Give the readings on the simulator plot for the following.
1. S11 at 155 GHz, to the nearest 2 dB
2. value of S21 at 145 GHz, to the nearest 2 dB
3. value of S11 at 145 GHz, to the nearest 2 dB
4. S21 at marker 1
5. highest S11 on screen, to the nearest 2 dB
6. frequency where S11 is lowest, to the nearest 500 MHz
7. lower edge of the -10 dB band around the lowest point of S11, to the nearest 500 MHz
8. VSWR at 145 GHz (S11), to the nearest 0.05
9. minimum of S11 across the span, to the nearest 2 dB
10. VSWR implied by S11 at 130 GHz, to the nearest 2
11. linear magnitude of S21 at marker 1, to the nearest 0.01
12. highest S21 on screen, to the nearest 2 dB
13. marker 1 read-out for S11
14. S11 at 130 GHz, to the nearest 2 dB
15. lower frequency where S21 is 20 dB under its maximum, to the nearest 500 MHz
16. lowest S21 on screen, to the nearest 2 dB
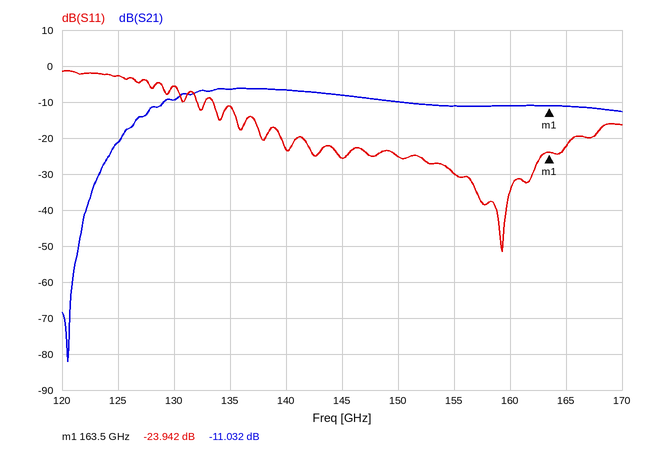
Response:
-30 dB
-8 dB
-26 dB
-11.032 dB
-2 dB
159.5 GHz
133.5 GHz
1.10
-52 dB
4
0.28
-6 dB
-23.942 dB
-6 dB
124.0 GHz
-82 dB
